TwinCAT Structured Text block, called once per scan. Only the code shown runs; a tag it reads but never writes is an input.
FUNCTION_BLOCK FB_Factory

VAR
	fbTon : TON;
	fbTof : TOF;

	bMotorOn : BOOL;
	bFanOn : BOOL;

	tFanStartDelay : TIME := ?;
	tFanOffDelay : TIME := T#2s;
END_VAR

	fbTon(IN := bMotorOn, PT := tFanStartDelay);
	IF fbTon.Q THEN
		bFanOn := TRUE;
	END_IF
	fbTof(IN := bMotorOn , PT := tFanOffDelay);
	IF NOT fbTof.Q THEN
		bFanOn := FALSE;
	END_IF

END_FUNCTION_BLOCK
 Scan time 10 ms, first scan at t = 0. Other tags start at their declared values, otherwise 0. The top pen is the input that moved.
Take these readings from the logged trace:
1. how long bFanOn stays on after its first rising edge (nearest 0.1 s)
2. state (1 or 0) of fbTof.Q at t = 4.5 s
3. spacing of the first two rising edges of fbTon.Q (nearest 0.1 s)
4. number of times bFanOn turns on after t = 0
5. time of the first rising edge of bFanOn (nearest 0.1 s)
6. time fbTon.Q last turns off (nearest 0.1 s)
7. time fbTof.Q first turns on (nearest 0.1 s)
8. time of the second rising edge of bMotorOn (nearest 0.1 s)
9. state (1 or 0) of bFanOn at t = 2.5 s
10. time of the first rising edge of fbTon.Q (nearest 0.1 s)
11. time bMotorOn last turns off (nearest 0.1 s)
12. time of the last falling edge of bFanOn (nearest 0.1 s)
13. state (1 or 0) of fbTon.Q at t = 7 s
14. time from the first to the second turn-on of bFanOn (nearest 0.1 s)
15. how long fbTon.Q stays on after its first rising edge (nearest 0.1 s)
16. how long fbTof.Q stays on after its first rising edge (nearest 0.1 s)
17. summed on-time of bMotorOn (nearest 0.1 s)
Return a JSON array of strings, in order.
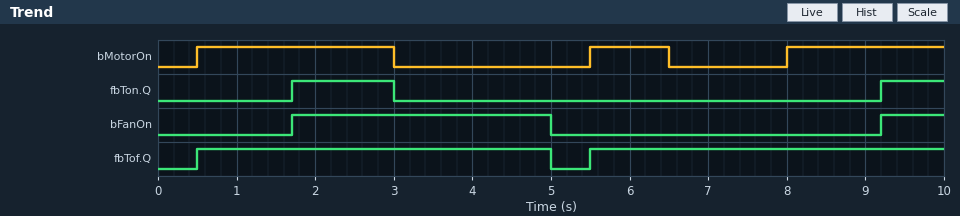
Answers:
["3.3 s", "1", "7.5 s", "2", "1.7 s", "3.0 s", "0.5 s", "5.5 s", "1", "1.7 s", "6.5 s", "5.0 s", "0", "7.5 s", "1.3 s", "4.5 s", "5.5 s"]
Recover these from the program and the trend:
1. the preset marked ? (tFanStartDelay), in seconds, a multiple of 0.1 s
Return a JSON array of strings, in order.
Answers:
["1.2 s"]
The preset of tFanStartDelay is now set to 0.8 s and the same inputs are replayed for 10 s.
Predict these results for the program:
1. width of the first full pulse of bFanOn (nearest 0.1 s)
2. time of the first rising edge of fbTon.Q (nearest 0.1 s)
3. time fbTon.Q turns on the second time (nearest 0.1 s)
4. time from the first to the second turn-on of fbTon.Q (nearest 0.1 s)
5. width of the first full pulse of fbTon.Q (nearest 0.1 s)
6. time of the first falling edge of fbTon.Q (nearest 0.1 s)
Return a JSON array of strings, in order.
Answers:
["3.7 s", "1.3 s", "6.3 s", "5.0 s", "1.7 s", "3.0 s"]
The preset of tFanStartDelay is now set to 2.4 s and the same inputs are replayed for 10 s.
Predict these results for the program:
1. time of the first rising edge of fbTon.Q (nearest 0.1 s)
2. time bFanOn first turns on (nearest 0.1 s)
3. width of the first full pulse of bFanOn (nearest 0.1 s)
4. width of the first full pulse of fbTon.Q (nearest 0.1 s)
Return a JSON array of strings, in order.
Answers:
["2.9 s", "2.9 s", "2.1 s", "0.1 s"]
